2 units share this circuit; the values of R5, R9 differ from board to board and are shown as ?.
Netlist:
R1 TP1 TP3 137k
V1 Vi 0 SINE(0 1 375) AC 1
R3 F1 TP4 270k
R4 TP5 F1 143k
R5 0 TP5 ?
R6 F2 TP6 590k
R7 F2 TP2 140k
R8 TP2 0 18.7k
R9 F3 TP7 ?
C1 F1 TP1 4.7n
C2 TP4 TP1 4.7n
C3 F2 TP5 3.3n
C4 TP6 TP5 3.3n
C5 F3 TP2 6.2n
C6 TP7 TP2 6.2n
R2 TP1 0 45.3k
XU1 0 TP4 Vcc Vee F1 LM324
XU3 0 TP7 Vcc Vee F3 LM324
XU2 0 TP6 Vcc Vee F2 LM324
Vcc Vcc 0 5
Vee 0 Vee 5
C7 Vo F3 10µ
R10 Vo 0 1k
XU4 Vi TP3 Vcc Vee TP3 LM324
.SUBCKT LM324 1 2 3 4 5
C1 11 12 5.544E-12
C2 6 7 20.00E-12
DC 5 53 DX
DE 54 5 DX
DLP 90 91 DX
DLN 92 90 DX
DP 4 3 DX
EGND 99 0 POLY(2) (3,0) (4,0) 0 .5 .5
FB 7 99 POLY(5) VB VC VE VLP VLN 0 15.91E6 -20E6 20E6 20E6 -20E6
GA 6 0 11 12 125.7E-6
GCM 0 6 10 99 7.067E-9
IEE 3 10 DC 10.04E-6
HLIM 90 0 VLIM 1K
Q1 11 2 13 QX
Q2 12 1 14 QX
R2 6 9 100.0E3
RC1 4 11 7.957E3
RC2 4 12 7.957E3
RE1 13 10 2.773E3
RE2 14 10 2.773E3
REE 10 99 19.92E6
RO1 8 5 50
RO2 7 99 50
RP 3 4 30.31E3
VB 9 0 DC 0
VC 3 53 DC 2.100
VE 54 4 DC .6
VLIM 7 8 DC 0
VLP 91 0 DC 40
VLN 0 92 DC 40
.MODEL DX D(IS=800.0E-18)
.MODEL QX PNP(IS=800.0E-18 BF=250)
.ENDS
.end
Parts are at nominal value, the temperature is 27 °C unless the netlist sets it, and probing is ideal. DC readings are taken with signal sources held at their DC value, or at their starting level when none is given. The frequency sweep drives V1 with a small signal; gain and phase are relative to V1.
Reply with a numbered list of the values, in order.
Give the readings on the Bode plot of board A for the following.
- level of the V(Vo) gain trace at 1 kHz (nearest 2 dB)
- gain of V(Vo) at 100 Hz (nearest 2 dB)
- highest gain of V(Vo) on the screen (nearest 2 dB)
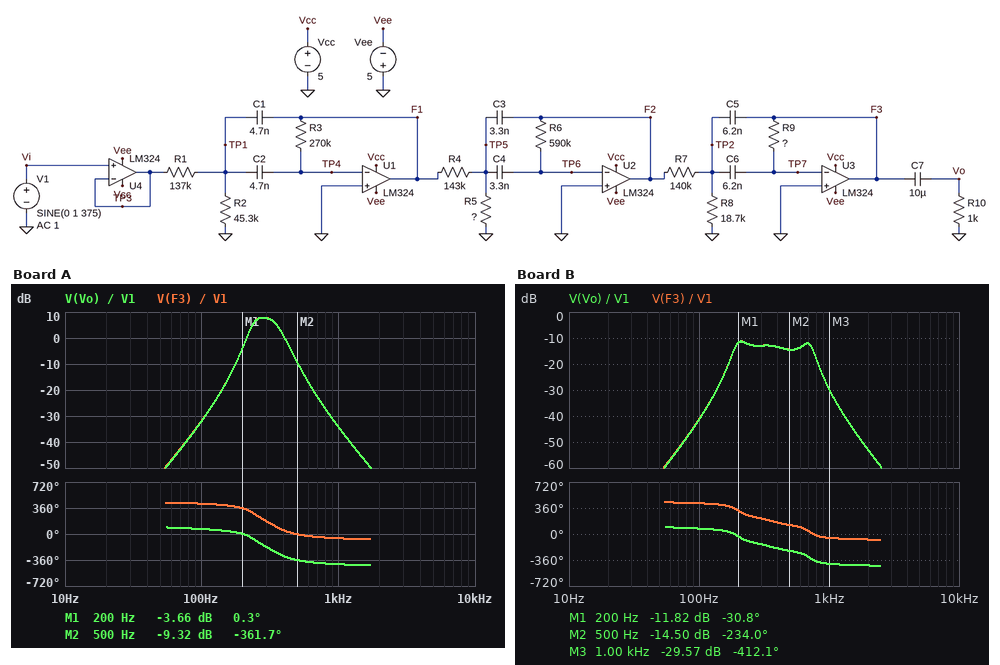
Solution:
1. -34 dB
2. -32 dB
3. 8 dB
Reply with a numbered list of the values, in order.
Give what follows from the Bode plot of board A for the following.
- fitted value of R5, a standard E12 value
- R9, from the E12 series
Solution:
1. 47 kΩ
2. 680 kΩ
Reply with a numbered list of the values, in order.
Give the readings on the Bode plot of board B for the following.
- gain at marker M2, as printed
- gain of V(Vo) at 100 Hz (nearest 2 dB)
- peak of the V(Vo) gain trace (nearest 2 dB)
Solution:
1. -14.50 dB
2. -42 dB
3. -12 dB
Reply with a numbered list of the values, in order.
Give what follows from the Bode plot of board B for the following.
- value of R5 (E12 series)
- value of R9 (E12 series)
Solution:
1. 8.2 kΩ
2. 1 MΩ
